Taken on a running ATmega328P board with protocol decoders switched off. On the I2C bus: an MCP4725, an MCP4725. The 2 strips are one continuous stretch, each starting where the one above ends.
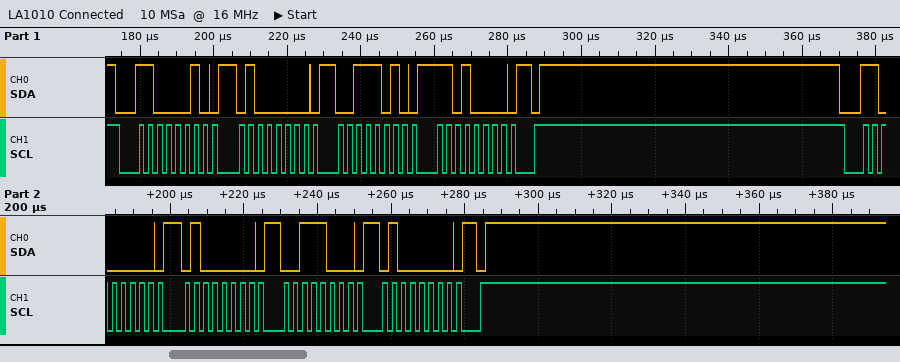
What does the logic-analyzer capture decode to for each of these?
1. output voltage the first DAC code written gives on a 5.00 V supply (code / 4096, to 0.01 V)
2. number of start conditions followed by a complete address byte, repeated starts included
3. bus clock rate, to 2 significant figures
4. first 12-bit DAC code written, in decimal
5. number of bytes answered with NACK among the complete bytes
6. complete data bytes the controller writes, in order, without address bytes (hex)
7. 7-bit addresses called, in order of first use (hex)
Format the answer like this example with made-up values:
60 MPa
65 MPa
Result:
1.15 V
2
400 kHz
941
0
40 3A D0 40 38 40
0x61 0x60
